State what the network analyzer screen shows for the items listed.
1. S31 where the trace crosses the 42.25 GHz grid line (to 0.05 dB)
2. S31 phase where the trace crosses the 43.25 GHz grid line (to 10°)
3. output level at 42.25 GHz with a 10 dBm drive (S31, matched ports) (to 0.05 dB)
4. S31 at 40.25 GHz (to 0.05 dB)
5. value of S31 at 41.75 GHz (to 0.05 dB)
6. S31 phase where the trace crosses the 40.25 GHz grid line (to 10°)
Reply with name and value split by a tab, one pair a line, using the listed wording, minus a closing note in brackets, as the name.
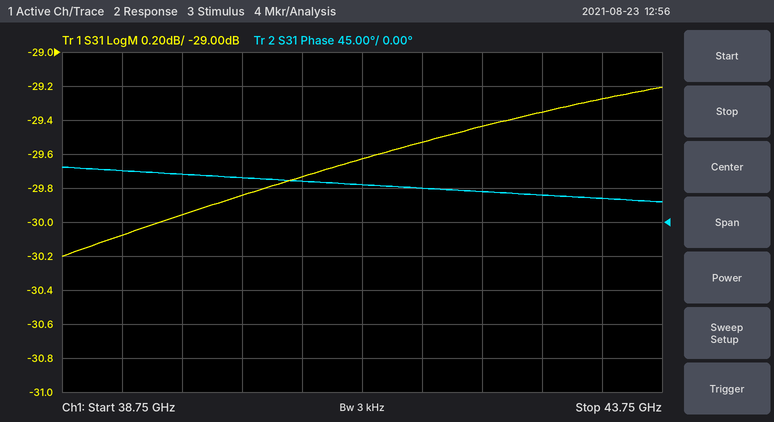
S31 where the trace crosses the 42.25 GHz grid line	-29.45 dB
S31 phase where the trace crosses the 43.25 GHz grid line	30°
output level at 42.25 GHz with a 10 dBm drive (S31, matched ports)	-19.45 dBm
S31 at 40.25 GHz	-29.85 dB
value of S31 at 41.75 GHz	-29.55 dB
S31 phase where the trace crosses the 40.25 GHz grid line	60°
